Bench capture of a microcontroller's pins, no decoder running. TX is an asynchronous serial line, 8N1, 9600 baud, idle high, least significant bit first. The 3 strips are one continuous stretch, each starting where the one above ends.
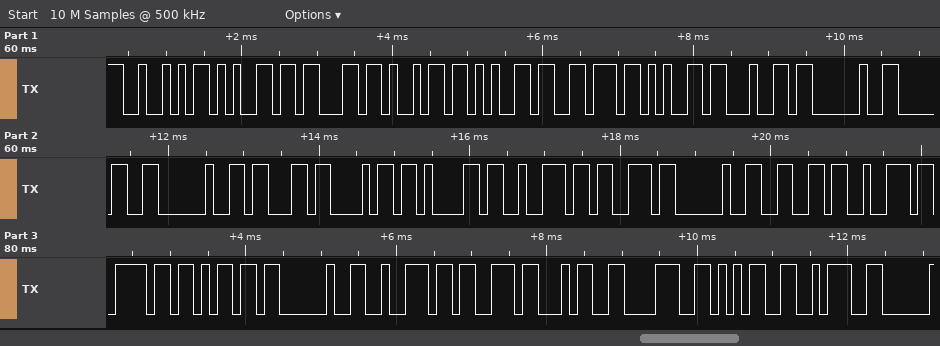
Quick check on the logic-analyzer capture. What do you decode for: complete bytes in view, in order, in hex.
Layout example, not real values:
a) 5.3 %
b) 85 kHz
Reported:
a) 52 65 63 69 65 76 65 64 20 30 20 63 68 61 72 73 20 66 72 6F 6D 20 72 73 34 38 35 3A
